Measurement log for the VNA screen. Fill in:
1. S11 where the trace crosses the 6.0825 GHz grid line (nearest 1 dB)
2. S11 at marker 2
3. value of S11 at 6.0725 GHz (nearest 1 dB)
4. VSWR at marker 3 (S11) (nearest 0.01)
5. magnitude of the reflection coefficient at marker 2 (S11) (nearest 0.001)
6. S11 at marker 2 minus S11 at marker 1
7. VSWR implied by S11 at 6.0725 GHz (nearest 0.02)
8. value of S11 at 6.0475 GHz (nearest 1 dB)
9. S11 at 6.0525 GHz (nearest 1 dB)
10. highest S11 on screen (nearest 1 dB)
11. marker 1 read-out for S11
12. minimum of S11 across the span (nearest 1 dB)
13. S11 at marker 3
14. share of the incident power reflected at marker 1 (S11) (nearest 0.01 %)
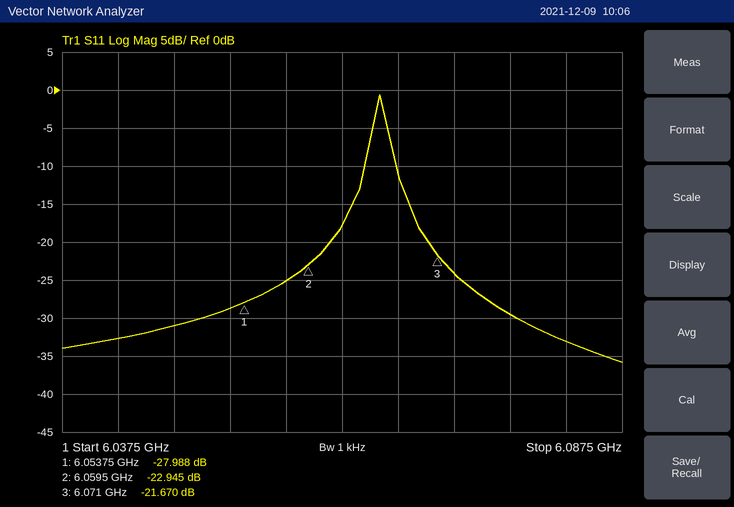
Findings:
-33 dB
-22.945 dB
-24 dB
1.18
0.071
5.043 dB
1.14
-31 dB
-29 dB
-1 dB
-27.988 dB
-36 dB
-21.670 dB
0.16 %
